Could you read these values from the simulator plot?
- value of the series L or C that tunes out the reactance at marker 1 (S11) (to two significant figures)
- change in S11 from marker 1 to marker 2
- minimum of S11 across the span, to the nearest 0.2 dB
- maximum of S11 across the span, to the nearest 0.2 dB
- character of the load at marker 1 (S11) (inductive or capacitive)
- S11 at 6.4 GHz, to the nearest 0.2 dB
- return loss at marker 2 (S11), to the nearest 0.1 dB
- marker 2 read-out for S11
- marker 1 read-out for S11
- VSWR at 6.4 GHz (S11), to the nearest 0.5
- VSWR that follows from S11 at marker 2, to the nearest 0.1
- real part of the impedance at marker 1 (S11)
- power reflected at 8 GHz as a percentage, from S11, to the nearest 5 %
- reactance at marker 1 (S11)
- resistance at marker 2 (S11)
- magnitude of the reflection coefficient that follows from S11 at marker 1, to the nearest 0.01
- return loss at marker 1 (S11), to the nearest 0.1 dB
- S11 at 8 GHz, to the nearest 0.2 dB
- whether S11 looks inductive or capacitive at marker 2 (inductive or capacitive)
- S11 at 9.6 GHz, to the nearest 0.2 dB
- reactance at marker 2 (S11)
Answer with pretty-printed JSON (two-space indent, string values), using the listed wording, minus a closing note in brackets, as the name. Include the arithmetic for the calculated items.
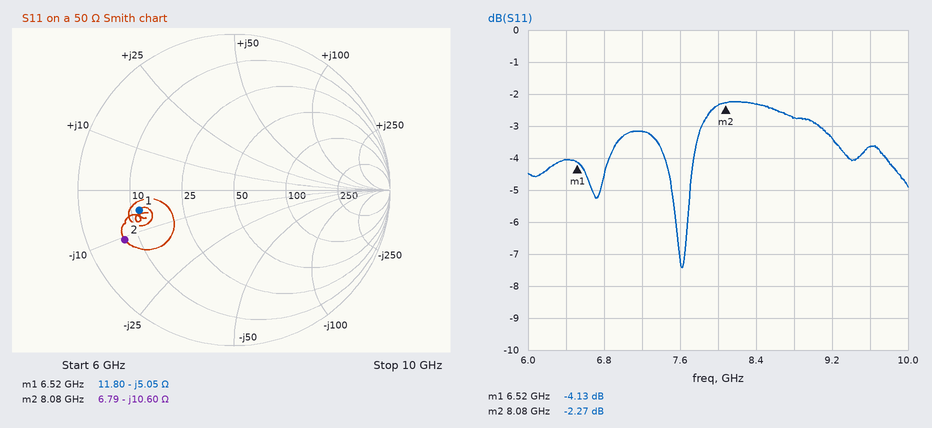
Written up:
{
  "value of the series L or C that tunes out the reactance at marker 1 (S11)": "L = 5.05 Ω/(2π × 6.52 GHz) ≈ 123 pH, so 120 pH to two significant figures",
  "change in S11 from marker 1 to marker 2": "-2.27 − (-4.13) = 1.86 dB",
  "minimum of S11 across the span, to the nearest 0.2 dB": "-7.4 dB",
  "maximum of S11 across the span, to the nearest 0.2 dB": "-2.2 dB",
  "character of the load at marker 1 (S11)": "capacitive",
  "S11 at 6.4 GHz, to the nearest 0.2 dB": "-4.0 dB",
  "return loss at marker 2 (S11), to the nearest 0.1 dB": "2.3 dB",
  "marker 2 read-out for S11": "-2.27 dB",
  "marker 1 read-out for S11": "-4.13 dB",
  "VSWR at 6.4 GHz (S11), to the nearest 0.5": "|Γ| = 10^(-4/20) = 0.6310; VSWR = (1 + 0.6310)/(1 − 0.6310) ≈ 4.42, so 4.5 to the nearest 0.5",
  "VSWR that follows from S11 at marker 2, to the nearest 0.1": "(1 + 0.7700)/(1 − 0.7700) ≈ 7.7",
  "real part of the impedance at marker 1": "11.80 Ω",
  "power reflected at 8 GHz as a percentage, from S11, to the nearest 5 %": "10^(-2.4/10) ≈ 57.5 %, so 60 % to the nearest 5 %",
  "reactance at marker 1": "-5.05 Ω",
  "resistance at marker 2": "6.79 Ω",
  "magnitude of the reflection coefficient that follows from S11 at marker 1, to the nearest 0.01": "10^(-4.13/20) ≈ 0.62",
  "return loss at marker 1 (S11), to the nearest 0.1 dB": "4.1 dB",
  "S11 at 8 GHz, to the nearest 0.2 dB": "-2.4 dB",
  "whether S11 looks inductive or capacitive at marker 2": "capacitive",
  "S11 at 9.6 GHz, to the nearest 0.2 dB": "-3.6 dB",
  "reactance at marker 2": "-10.60 Ω"
}
